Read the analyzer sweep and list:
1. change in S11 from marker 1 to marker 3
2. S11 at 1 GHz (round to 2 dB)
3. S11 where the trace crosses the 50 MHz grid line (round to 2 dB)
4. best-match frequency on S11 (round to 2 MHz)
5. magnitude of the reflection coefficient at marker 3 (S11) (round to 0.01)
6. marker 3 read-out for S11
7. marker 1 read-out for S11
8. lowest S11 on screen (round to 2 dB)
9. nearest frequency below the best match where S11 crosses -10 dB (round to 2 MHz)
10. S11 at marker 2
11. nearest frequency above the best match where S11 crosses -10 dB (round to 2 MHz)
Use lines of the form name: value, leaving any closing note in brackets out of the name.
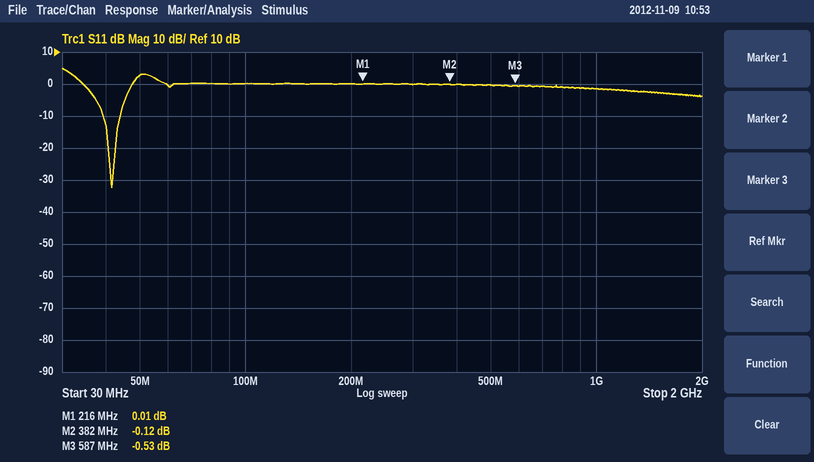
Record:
change in S11 from marker 1 to marker 3: -0.54 dB
S11 at 1 GHz: -2 dB
S11 where the trace crosses the 50 MHz grid line: 2 dB
best-match frequency on S11: 42 MHz
magnitude of the reflection coefficient at marker 3 (S11): 0.94
marker 3 read-out for S11: -0.53 dB
marker 1 read-out for S11: 0.01 dB
lowest S11 on screen: -32 dB
nearest frequency below the best match where S11 crosses -10 dB: 40 MHz
S11 at marker 2: -0.12 dB
nearest frequency above the best match where S11 crosses -10 dB: 44 MHz
